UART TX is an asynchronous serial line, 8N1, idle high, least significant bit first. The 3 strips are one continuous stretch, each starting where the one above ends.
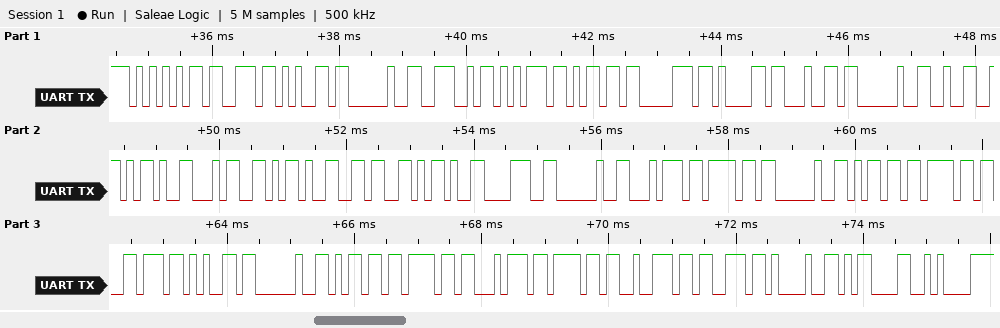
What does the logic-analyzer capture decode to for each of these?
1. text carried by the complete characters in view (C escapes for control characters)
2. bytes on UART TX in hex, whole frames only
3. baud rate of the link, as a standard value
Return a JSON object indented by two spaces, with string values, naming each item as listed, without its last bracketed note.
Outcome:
{
  "text carried by the complete characters in view": "\"Use Numpad 2-4-6-8 to move motors!\\r\\n\"",
  "bytes on UART TX in hex, whole frames only": "55 73 65 20 4E 75 6D 70 61 64 20 32 2D 34 2D 36 2D 38 20 74 6F 20 6D 6F 76 65 20 6D 6F 74 6F 72 73 21 0D 0A",
  "baud rate of the link, as a standard value": "9600 baud"
}
